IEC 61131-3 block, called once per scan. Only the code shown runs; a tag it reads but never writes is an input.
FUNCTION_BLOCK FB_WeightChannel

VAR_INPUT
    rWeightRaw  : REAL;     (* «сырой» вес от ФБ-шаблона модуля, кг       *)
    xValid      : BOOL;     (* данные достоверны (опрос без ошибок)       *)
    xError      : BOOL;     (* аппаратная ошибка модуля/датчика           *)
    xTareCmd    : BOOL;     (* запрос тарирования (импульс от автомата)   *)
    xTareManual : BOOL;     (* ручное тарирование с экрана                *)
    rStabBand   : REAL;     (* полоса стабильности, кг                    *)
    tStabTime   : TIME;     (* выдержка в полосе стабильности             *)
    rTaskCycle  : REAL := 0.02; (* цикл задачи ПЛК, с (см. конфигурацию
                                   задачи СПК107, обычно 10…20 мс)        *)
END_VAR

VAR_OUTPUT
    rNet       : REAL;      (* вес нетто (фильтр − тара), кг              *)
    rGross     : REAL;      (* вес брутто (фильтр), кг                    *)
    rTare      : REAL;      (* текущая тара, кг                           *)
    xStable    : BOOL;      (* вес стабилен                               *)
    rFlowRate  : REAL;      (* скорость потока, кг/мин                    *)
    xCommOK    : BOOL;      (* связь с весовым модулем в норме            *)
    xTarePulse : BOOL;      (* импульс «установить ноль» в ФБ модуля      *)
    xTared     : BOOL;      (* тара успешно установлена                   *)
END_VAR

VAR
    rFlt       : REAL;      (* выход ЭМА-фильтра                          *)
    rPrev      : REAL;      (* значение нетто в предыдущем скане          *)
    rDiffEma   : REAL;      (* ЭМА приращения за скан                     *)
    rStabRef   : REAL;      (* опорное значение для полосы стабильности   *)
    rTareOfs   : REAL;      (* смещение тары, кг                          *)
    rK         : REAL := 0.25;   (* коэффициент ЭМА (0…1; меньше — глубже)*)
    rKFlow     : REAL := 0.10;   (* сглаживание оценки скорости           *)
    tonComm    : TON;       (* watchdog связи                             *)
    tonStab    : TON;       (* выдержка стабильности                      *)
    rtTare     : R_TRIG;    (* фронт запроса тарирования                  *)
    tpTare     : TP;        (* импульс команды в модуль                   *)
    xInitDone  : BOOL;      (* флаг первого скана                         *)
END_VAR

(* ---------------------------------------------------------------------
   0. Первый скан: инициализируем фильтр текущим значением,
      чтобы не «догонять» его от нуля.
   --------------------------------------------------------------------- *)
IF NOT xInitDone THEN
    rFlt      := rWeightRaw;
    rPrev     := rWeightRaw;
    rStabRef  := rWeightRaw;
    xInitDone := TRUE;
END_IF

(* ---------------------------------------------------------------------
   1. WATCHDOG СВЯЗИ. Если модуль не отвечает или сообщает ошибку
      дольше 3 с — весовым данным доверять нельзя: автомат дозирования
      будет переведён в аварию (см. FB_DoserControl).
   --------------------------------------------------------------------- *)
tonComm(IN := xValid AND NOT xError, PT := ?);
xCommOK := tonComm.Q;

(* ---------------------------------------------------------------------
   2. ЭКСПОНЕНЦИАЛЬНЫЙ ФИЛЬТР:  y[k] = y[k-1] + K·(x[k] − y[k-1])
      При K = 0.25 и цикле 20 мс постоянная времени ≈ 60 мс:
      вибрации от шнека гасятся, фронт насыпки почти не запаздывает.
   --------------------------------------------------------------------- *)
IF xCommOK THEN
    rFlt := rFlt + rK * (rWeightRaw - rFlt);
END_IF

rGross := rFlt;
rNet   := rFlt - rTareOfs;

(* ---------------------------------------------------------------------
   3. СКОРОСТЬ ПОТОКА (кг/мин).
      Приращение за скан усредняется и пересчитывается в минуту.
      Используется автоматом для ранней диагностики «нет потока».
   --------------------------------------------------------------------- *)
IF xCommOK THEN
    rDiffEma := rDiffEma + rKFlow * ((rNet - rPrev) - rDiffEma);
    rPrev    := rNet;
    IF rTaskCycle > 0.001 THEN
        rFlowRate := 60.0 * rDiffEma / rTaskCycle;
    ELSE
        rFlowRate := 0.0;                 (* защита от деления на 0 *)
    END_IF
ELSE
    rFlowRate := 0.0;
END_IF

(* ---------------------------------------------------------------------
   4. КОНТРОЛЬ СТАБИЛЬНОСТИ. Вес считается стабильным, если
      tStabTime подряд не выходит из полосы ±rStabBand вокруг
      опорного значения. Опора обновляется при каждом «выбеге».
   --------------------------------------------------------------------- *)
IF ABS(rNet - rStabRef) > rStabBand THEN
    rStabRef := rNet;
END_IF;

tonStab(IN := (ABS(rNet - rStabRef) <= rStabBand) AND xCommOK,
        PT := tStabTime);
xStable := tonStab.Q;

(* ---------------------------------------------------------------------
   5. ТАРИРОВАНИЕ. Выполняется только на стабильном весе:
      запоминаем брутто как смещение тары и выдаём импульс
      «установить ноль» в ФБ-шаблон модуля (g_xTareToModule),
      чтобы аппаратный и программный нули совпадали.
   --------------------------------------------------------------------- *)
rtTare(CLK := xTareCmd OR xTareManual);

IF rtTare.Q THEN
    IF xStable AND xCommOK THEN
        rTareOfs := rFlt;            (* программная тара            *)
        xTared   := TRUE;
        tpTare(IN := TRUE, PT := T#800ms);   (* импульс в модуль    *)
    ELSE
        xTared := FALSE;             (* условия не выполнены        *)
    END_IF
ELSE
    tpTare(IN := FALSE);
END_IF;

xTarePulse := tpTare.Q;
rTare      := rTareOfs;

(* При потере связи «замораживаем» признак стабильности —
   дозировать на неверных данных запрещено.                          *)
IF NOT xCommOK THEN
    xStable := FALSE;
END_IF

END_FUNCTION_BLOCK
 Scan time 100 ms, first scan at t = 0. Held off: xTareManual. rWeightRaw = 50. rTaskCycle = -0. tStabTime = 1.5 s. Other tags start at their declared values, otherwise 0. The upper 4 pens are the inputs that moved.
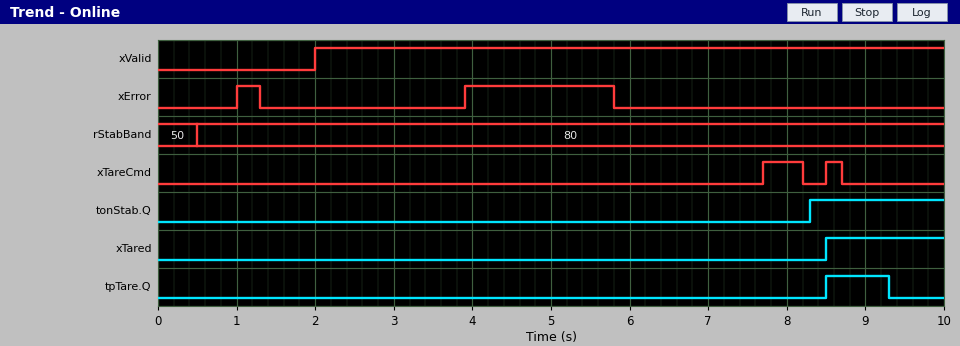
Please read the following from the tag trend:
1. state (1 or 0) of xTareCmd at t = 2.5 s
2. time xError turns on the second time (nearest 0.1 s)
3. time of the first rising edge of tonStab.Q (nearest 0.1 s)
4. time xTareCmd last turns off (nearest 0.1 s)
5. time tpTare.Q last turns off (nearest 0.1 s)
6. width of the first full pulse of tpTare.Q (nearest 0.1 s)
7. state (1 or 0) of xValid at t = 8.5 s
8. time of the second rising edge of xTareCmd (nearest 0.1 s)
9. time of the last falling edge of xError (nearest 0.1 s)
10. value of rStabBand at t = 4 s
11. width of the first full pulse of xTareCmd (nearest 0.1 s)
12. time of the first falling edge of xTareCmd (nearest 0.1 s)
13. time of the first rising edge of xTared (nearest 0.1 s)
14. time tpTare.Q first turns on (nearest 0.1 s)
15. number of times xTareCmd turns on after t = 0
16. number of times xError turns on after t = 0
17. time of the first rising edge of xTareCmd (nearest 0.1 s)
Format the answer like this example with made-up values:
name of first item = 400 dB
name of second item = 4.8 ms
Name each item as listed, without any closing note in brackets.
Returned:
state (1 or 0) of xTareCmd at t = 2.5 s = 0
time xError turns on the second time = 3.9 s
time of the first rising edge of tonStab.Q = 8.3 s
time xTareCmd last turns off = 8.7 s
time tpTare.Q last turns off = 9.3 s
width of the first full pulse of tpTare.Q = 0.8 s
state (1 or 0) of xValid at t = 8.5 s = 1
time of the second rising edge of xTareCmd = 8.5 s
time of the last falling edge of xError = 5.8 s
value of rStabBand at t = 4 s = 80
width of the first full pulse of xTareCmd = 0.5 s
time of the first falling edge of xTareCmd = 8.2 s
time of the first rising edge of xTared = 8.5 s
time tpTare.Q first turns on = 8.5 s
number of times xTareCmd turns on after t = 0 = 2
number of times xError turns on after t = 0 = 2
time of the first rising edge of xTareCmd = 7.7 s
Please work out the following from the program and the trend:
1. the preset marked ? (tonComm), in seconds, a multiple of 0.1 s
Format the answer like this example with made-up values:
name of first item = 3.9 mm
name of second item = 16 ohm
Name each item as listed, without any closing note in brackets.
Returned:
the preset marked ? (tonComm), in seconds, a multiple of 0.1 s = 1.0 s
